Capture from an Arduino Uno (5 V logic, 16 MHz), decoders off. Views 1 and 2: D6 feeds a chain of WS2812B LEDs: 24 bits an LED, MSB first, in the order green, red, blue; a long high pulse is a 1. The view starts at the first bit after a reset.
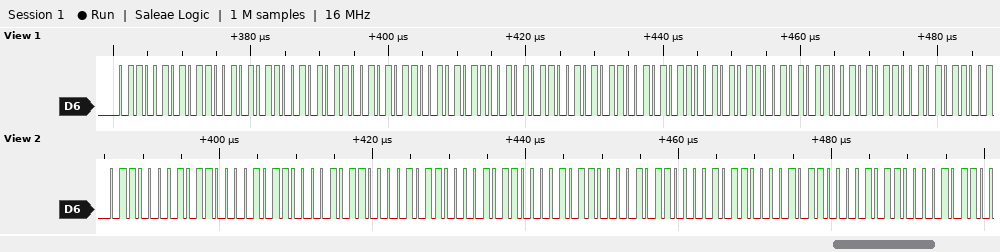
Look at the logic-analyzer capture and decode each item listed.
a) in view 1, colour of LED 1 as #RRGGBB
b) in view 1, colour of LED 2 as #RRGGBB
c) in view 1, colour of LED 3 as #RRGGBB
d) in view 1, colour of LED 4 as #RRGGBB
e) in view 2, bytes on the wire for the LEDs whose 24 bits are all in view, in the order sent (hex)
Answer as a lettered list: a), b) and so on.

a) #656565
b) #656565
c) #656565
d) #656565
e) 61 61 61 61 61 61 61 61 61
